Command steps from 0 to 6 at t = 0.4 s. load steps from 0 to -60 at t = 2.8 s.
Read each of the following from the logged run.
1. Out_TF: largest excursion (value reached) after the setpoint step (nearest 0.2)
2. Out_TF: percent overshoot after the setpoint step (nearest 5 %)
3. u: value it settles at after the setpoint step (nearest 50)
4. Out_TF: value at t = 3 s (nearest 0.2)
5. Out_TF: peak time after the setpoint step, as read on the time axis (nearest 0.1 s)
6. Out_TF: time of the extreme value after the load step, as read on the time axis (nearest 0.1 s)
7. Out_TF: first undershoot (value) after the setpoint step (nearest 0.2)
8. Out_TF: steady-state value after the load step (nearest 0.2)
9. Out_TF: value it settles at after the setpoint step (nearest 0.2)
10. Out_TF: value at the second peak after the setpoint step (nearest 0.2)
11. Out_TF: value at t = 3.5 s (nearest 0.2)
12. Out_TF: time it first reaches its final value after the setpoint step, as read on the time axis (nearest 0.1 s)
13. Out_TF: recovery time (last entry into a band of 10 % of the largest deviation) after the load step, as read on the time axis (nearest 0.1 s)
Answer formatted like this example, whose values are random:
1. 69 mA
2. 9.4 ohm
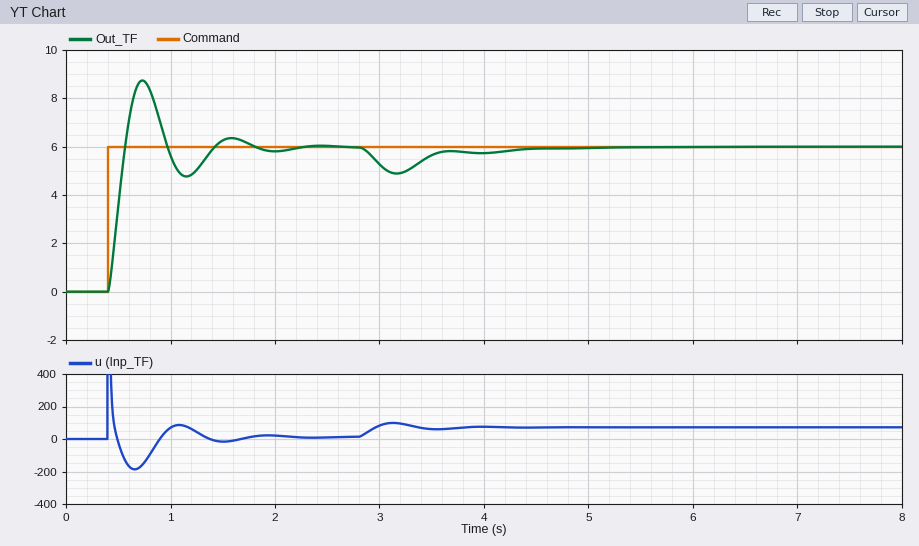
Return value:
1. 8.8
2. 45 %
3. 0
4. 5.2
5. 0.7 s
6. 3.2 s
7. 4.8
8. 6.0
9. 6.0
10. 6.4
11. 5.6
12. 0.6 s
13. 4.4 s
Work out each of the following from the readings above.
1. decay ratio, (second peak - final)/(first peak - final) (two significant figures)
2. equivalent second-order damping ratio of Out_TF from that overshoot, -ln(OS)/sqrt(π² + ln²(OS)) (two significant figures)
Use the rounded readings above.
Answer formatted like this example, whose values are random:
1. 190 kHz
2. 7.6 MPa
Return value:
1. 0.14
2. 0.25
